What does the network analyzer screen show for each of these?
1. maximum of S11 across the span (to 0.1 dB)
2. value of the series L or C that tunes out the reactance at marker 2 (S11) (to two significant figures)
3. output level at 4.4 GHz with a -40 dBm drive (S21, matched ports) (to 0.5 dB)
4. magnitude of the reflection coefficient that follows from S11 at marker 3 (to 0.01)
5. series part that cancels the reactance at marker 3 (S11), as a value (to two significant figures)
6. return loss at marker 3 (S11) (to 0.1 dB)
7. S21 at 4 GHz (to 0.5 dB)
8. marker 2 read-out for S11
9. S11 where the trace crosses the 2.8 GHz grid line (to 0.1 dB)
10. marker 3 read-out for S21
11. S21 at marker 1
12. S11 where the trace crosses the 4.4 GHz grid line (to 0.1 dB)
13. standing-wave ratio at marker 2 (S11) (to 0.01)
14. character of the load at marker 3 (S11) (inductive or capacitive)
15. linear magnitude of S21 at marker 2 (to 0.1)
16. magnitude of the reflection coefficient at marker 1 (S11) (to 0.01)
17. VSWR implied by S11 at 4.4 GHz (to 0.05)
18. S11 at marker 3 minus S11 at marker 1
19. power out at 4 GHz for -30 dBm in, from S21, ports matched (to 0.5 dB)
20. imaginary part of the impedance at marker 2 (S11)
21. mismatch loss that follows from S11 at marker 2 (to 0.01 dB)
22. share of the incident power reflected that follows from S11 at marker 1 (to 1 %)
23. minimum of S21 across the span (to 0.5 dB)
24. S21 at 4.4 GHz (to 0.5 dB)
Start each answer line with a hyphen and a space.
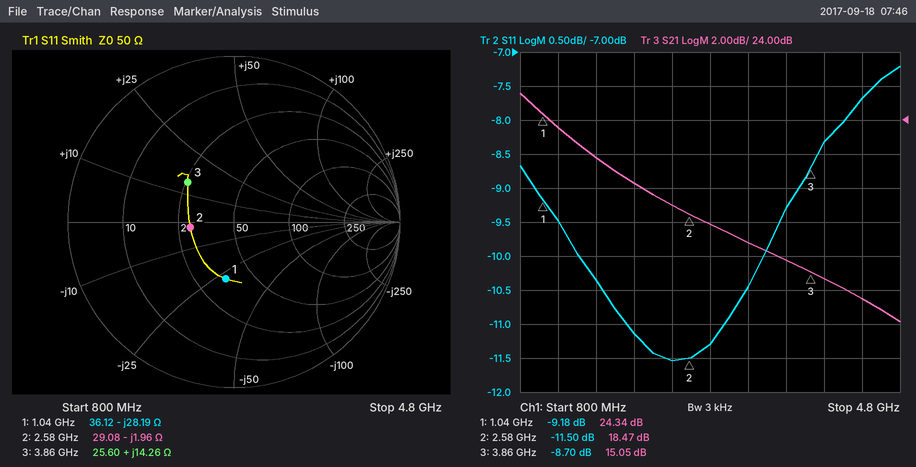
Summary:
- -7.2 dB
- 120 pH
- -26.5 dBm
- 0.37
- 2.9 pF
- 8.7 dB
- 14.5 dB
- -11.50 dB
- -11.3 dB
- 15.05 dB
- 24.34 dB
- -7.7 dB
- 1.72
- inductive
- 8.4
- 0.35
- 2.40
- 0.48 dB
- -15.5 dBm
- -1.96 Ω
- 0.32 dB
- 12 %
- 12.0 dB
- 13.5 dB
